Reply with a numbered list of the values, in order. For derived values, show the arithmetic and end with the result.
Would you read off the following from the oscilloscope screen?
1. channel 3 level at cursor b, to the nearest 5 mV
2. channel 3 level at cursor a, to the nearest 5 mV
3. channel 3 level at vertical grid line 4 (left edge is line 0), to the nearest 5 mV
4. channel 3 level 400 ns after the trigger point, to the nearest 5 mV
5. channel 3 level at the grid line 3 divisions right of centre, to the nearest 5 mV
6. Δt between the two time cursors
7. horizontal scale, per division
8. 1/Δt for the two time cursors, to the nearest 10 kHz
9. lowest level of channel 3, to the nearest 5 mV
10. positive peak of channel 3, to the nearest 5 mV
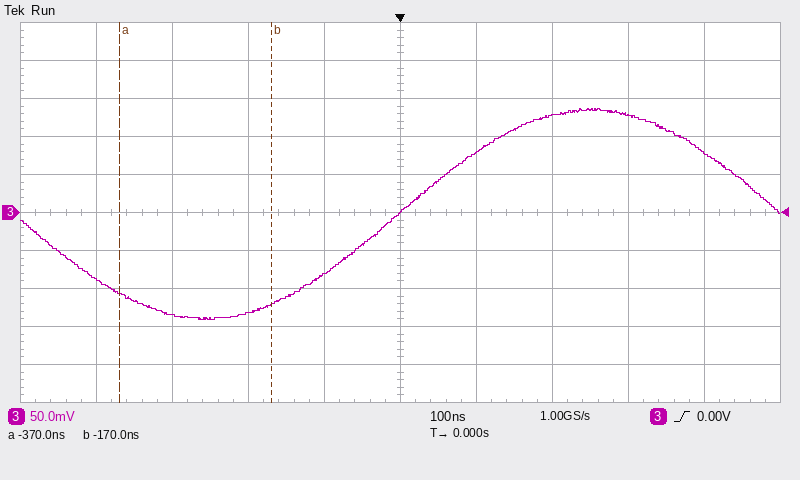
1. -120 mV
2. -105 mV
3. -80 mV
4. 80 mV
5. 130 mV
6. -170 ns − (-370 ns) = 200 ns
7. 100 ns
8. 1 / 200 ns ≈ 5.00 MHz
9. -140 mV
10. 135 mV
